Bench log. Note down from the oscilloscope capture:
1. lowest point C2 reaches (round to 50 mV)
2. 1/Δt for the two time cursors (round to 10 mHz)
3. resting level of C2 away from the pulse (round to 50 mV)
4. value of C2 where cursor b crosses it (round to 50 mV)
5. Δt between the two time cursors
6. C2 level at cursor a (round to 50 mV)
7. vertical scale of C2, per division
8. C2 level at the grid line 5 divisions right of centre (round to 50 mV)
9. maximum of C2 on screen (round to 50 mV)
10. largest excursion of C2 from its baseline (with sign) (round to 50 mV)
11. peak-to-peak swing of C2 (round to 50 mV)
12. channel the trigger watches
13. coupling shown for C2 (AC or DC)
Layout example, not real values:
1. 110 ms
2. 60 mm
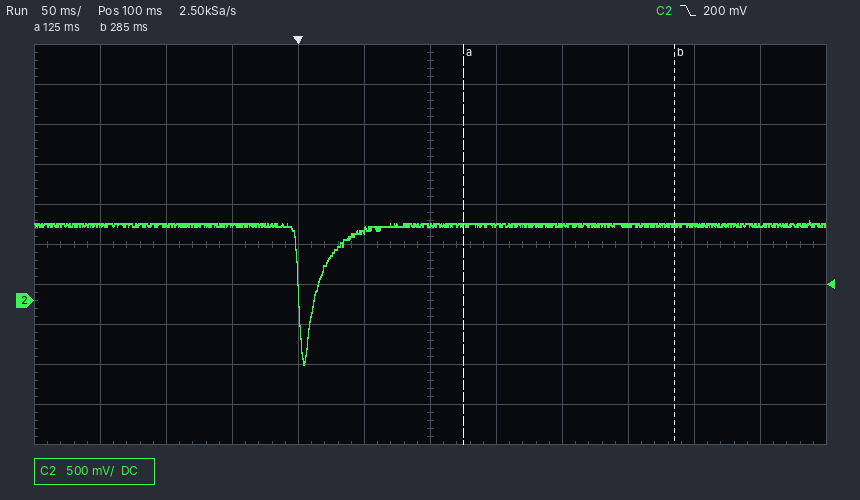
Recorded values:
1. -800 mV
2. 6.25 Hz
3. 950 mV
4. 950 mV
5. 160 ms
6. 950 mV
7. 500 mV
8. 950 mV
9. 1.00 V
10. -1.75 V
11. 1.80 V
12. C2
13. DC
